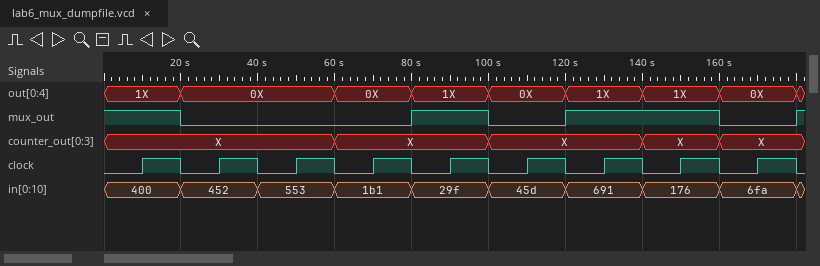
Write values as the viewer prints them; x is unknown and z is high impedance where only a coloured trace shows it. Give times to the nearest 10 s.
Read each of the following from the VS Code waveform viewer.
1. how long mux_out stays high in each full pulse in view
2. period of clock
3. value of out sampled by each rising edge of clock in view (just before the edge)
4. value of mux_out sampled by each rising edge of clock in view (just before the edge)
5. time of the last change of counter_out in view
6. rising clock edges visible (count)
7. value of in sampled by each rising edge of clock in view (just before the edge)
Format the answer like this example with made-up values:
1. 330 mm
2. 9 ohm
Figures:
1. 20 s, 40 s
2. 20 s
3. 1X, 0X, 0X, 0X, 1X, 0X, 1X, 1X, 0X
4. 1 0 0 0 1 0 1 1 0
5. 160 s
6. 9
7. 400, 452, 553, 1b1, 29f, 45d, 691, 176, 6fa
